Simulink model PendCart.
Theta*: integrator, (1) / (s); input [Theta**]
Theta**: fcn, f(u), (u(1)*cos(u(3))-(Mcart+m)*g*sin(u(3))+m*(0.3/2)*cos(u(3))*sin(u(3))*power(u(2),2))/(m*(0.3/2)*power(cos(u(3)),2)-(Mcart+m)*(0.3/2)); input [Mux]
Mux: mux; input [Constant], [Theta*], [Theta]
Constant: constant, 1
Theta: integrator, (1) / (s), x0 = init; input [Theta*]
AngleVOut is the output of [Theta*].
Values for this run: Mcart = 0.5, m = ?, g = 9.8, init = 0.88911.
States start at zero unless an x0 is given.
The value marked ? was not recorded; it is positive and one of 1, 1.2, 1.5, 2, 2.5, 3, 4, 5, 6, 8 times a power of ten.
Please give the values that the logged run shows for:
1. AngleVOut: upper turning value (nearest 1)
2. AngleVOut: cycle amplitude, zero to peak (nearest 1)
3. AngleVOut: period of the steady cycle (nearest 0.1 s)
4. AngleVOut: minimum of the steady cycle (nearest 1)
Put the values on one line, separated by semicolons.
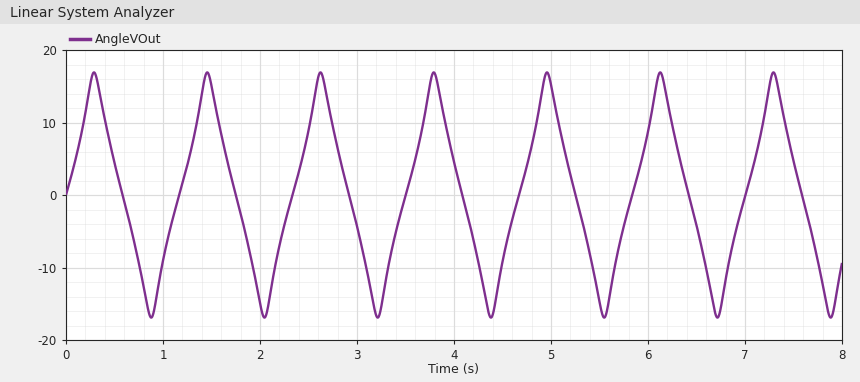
17; 17; 1.2 s; -17
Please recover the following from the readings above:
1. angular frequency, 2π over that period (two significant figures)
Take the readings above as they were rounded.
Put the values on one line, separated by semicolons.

5.2 rad/s
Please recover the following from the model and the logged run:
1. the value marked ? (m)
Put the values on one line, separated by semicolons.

0.12
